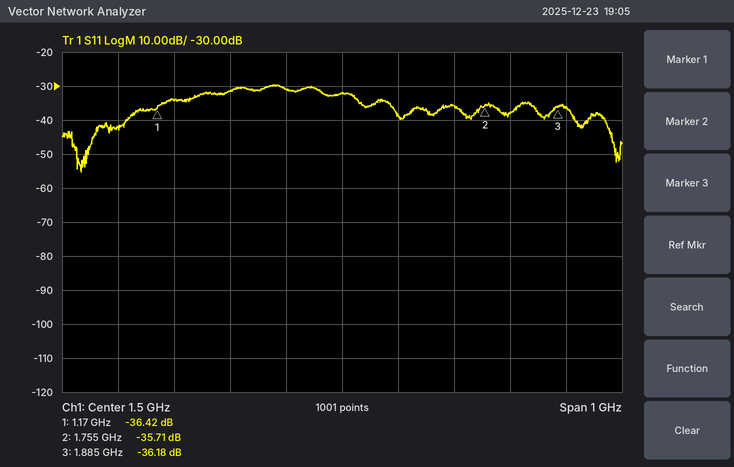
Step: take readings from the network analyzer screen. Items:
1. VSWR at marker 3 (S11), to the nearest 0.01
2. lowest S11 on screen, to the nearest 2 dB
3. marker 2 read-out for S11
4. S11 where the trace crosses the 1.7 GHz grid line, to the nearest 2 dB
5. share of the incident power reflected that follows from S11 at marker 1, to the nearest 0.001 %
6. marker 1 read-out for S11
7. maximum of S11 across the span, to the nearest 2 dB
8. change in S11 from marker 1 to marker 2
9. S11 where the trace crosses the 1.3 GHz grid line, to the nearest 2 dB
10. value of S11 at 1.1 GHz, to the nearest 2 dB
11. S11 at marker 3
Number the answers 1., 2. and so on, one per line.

1. 1.03
2. -56 dB
3. -35.71 dB
4. -36 dB
5. 0.023 %
6. -36.42 dB
7. -30 dB
8. 0.71 dB
9. -32 dB
10. -42 dB
11. -36.18 dB
